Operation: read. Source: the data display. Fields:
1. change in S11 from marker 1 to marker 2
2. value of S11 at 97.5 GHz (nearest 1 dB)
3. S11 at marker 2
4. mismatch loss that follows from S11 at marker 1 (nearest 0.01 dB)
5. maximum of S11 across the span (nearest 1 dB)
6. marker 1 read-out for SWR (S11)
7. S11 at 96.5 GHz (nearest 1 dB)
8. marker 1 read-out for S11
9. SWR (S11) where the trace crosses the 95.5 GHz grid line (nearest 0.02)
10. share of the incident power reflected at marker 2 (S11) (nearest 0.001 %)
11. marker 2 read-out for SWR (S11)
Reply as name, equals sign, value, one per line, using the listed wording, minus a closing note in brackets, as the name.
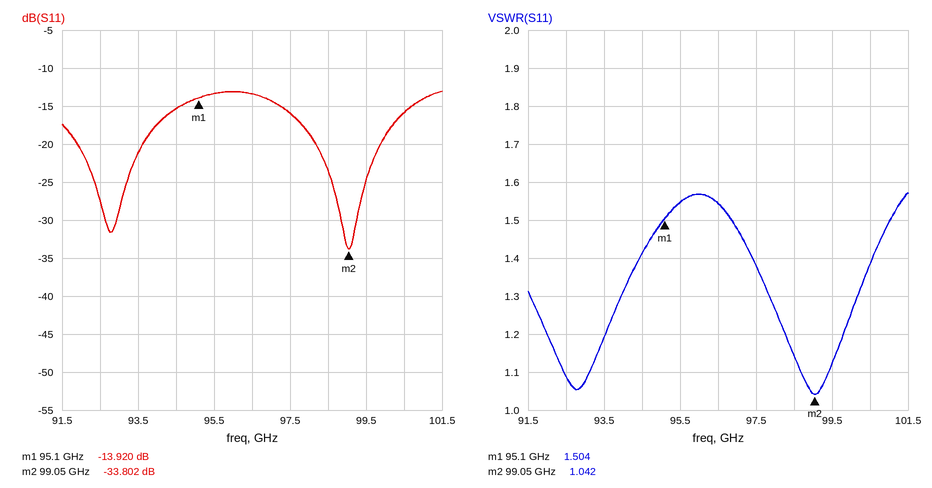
change in S11 from marker 1 to marker 2 = -19.882 dB
value of S11 at 97.5 GHz = -16 dB
S11 at marker 2 = -33.802 dB
mismatch loss that follows from S11 at marker 1 = 0.18 dB
maximum of S11 across the span = -13 dB
marker 1 read-out for SWR = 1.504
S11 at 96.5 GHz = -13 dB
marker 1 read-out for S11 = -13.920 dB
SWR (S11) where the trace crosses the 95.5 GHz grid line = 1.54
share of the incident power reflected at marker 2 (S11) = 0.042 %
marker 2 read-out for SWR = 1.042
